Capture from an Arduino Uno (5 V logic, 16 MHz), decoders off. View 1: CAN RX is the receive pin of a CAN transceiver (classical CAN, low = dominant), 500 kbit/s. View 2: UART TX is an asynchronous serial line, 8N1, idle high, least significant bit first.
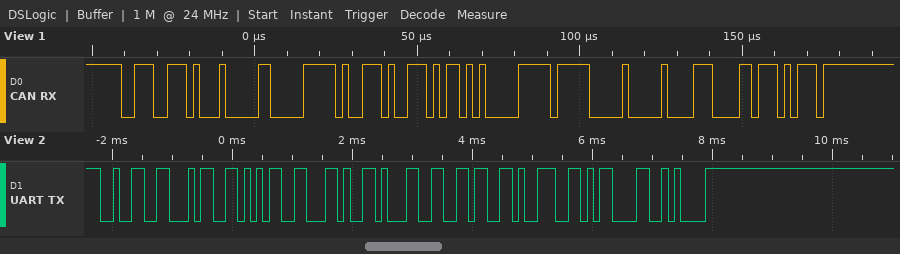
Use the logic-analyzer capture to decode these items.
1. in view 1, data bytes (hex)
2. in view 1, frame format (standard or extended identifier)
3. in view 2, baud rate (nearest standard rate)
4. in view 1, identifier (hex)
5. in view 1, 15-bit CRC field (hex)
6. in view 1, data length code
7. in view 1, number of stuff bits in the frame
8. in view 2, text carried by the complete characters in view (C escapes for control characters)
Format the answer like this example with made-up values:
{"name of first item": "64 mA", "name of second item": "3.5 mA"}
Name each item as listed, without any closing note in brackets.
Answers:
{"in view 1, data bytes": "20 F9 D3 AD 41 FF 00 07", "in view 1, frame format": "standard", "in view 2, baud rate": "9600 baud", "in view 1, identifier": "0x39D", "in view 1, 15-bit CRC field": "0x06EB", "in view 1, data length code": "8", "in view 1, number of stuff bits in the frame": "8", "in view 2, text carried by the complete characters in view": "\"245,169\\r\\n\""}
